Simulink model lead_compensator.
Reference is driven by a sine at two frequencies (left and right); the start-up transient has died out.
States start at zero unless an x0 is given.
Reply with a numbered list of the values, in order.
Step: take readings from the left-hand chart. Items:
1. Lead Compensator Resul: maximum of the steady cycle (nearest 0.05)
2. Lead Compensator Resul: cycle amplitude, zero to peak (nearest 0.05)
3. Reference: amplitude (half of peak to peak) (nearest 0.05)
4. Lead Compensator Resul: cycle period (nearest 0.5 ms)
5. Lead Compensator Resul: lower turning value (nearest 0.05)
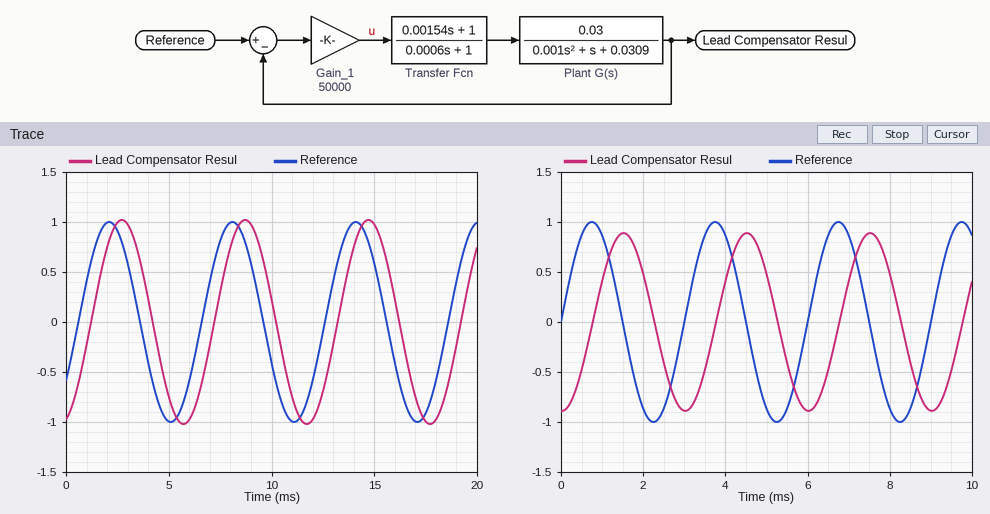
1. 1.00
2. 1.00
3. 1.00
4. 6.0 ms
5. -1.00
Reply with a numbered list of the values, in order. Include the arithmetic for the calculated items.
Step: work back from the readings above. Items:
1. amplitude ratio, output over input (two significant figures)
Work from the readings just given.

1. 1 / 1 = 1.0
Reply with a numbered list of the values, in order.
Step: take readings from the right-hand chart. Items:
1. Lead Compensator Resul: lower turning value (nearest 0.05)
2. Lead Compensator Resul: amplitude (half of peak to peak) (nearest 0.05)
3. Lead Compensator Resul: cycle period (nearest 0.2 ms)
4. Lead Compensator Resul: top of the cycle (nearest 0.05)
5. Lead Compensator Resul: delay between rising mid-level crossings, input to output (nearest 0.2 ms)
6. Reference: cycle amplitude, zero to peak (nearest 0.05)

1. -0.90
2. 0.90
3. 3.0 ms
4. 0.90
5. 0.8 ms
6. 1.00
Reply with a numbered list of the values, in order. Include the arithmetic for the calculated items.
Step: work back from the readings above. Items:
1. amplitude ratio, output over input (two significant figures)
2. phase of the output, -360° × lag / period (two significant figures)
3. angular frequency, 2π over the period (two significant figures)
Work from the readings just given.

1. 0.9 / 1 = 0.90
2. -360 × 0.8 / 3 = -96°
3. 2π / 3 = 2.1 rad/ms
